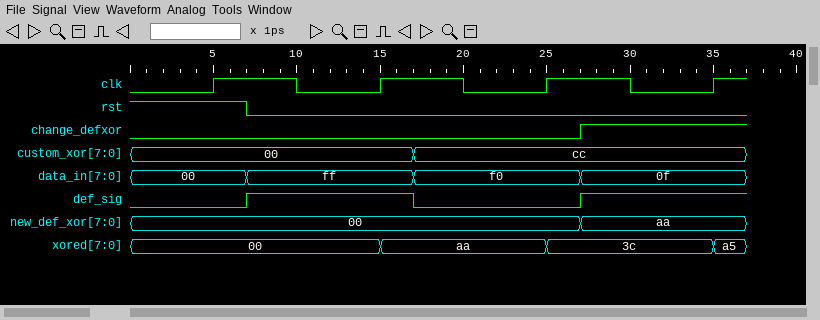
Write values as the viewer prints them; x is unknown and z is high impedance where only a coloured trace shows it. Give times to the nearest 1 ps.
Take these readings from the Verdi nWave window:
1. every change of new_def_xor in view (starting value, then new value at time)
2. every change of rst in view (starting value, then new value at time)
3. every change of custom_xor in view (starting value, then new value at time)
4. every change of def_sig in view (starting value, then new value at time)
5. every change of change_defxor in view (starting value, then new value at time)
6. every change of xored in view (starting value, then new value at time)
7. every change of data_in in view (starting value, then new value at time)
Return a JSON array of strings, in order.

["00, aa at 27 ps", "1, 0 at 7 ps", "00, cc at 17 ps", "0, 1 at 7 ps, 0 at 17 ps, 1 at 27 ps", "0, 1 at 27 ps", "00, aa at 15 ps, 3c at 25 ps, a5 at 35 ps", "00, ff at 7 ps, f0 at 17 ps, 0f at 27 ps"]
